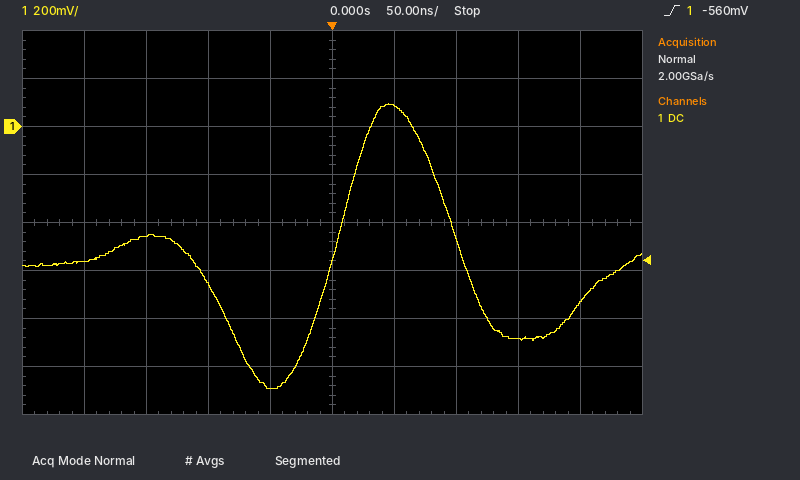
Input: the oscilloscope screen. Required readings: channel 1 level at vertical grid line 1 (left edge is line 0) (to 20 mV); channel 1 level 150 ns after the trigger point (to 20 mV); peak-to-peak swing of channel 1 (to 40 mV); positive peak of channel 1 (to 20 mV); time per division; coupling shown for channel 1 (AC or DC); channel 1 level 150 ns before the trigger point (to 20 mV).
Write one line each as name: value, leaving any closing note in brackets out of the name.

channel 1 level at vertical grid line 1 (left edge is line 0): -560 mV
channel 1 level 150 ns after the trigger point: -880 mV
peak-to-peak swing of channel 1: 1.20 V
positive peak of channel 1: 100 mV
time per division: 50 ns
coupling shown for channel 1: DC
channel 1 level 150 ns before the trigger point: -460 mV
